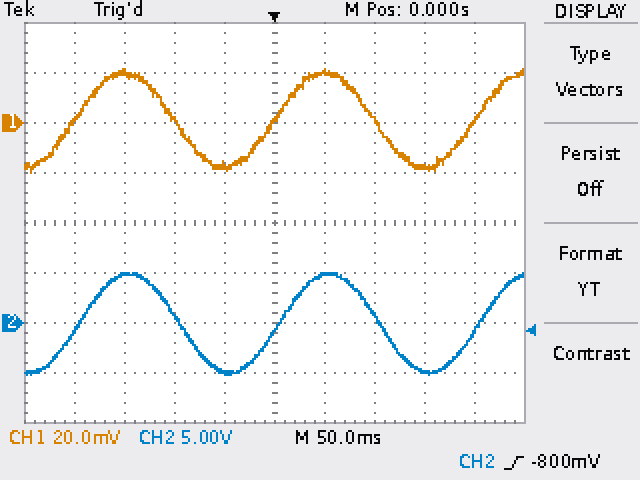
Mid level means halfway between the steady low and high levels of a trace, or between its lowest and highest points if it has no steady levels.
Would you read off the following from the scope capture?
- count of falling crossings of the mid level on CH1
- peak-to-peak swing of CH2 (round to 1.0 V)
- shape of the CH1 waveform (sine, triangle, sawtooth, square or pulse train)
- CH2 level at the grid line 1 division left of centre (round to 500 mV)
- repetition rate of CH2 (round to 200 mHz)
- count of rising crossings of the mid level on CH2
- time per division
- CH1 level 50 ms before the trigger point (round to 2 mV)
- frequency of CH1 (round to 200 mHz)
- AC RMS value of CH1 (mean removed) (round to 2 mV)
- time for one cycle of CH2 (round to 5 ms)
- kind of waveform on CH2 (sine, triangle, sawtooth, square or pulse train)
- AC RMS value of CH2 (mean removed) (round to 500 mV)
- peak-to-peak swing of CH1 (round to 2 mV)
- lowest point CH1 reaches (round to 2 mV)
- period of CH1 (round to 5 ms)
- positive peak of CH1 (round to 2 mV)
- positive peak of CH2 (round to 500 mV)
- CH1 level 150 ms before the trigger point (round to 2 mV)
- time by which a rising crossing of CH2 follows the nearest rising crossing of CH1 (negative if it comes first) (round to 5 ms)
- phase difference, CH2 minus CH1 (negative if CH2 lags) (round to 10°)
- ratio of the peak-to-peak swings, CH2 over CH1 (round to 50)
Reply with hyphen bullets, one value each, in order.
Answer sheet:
- 2
- 10.0 V
- sine
- -5.0 V
- 5.0 Hz
- 3
- 50 ms
- -18 mV
- 5.0 Hz
- 14 mV
- 200 ms
- sine
- 3.5 V
- 42 mV
- -20 mV
- 200 ms
- 22 mV
- 5.0 V
- 20 mV
- +5 ms
- -10°
- 250
